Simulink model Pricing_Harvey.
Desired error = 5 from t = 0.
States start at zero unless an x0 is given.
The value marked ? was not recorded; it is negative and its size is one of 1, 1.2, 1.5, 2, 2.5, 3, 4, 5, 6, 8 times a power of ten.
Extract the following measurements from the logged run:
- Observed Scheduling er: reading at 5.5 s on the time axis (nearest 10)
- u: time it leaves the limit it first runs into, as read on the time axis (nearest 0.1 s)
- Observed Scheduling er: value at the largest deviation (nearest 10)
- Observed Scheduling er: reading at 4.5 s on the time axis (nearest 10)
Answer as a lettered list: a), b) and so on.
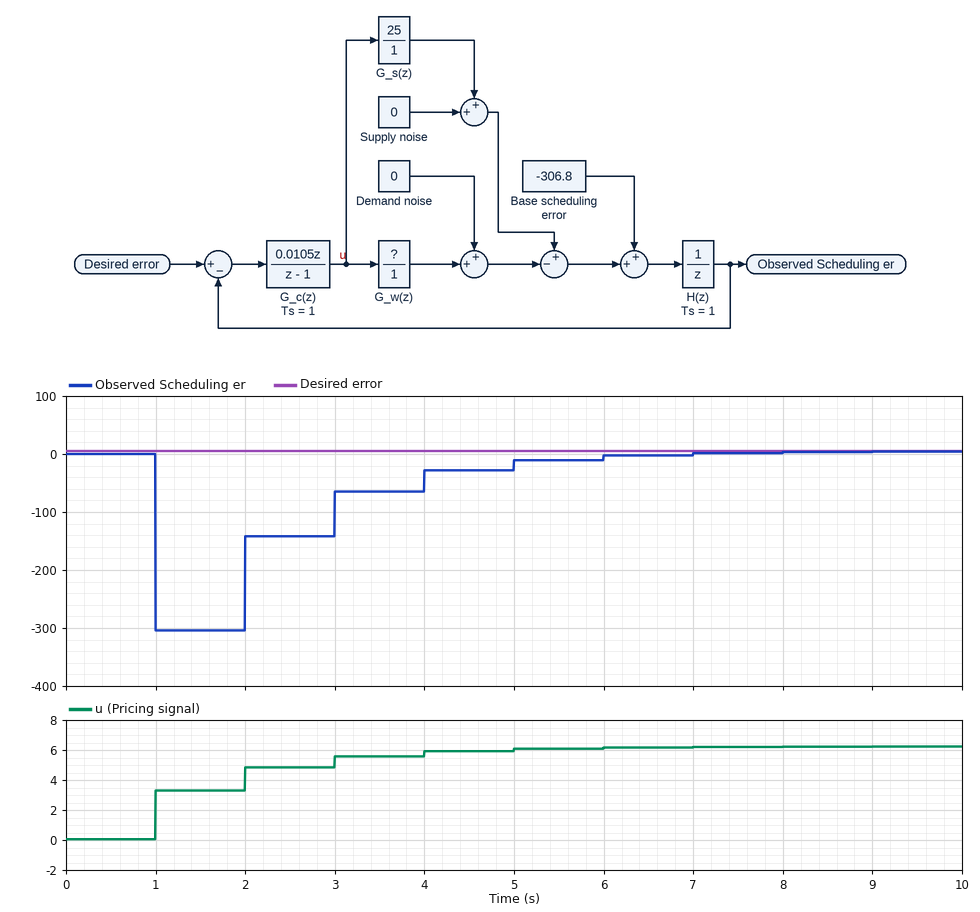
a) -10
b) 1.0 s
c) -300
d) -30
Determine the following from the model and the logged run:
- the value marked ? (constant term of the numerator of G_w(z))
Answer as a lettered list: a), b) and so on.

a) -25
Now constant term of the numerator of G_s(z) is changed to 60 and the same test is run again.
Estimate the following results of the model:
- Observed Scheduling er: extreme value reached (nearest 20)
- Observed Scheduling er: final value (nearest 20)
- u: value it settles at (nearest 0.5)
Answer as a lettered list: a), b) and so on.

a) -300
b) 0
c) 3.5
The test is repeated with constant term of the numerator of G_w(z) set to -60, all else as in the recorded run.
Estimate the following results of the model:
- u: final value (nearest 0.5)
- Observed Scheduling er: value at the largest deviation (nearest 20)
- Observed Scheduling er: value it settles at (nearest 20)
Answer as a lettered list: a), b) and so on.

a) 3.5
b) -300
c) 0
